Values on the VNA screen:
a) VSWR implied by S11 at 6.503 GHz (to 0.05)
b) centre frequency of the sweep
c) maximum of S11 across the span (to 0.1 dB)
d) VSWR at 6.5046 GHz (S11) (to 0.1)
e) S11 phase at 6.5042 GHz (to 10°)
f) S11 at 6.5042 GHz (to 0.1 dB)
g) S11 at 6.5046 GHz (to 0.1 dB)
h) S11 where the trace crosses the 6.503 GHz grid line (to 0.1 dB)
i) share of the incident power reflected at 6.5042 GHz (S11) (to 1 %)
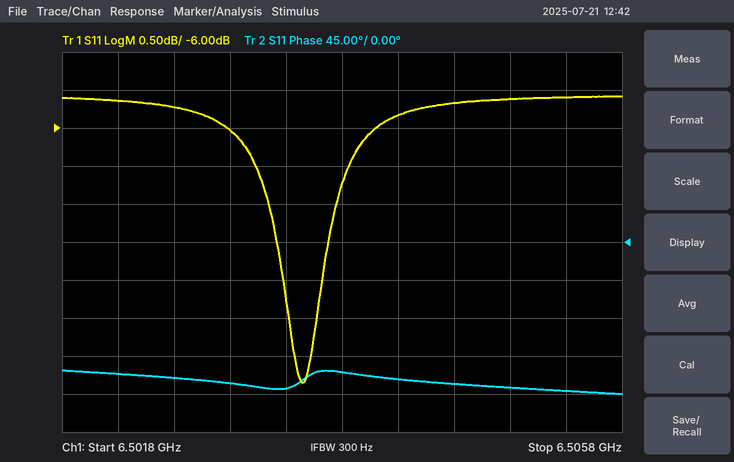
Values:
3.00
6.5038 GHz
-5.6 dB
3.2
-160°
-5.8 dB
-5.7 dB
-6.0 dB
26 %
